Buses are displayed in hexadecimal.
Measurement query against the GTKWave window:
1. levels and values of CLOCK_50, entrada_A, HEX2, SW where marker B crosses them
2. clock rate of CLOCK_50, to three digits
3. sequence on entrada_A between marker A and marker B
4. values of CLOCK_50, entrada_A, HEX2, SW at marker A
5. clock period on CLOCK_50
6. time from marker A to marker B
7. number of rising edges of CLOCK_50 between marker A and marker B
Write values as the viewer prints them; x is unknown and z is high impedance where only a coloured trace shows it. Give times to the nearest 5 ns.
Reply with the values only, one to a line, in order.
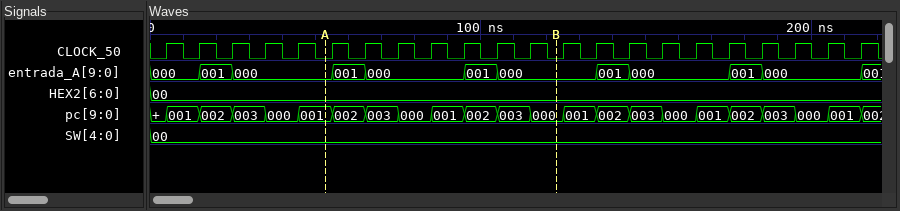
CLOCK_50=0, entrada_A=000, HEX2=00, SW=00
100 MHz
000, 001, 000, 001, 000
CLOCK_50=0, entrada_A=000, HEX2=00, SW=00
10 ns
70 ns
7
